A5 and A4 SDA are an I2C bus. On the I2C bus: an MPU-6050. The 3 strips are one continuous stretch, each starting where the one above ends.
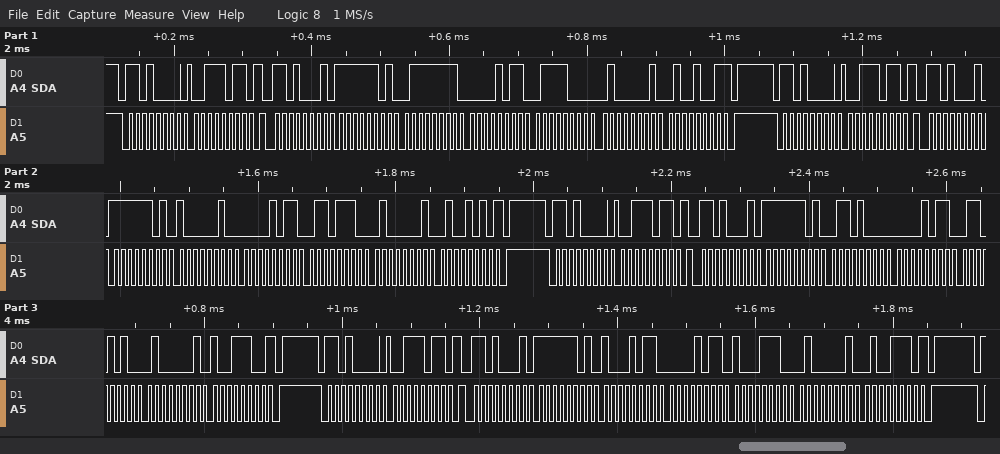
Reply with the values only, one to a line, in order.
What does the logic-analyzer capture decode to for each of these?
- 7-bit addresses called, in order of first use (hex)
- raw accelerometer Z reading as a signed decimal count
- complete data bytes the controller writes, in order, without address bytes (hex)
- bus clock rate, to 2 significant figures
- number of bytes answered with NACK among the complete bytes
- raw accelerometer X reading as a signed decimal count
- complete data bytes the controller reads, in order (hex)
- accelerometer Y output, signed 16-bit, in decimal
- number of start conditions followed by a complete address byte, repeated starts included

0x68
16713
3B 3B 3B 3B
100 kHz
4
-641
FD 7F 0B 78 41 49 FD 82 0B 6E 41 4A FD 68 0B 6A 41 9C FD 8B 0B 8E 41 4E
2936
8
